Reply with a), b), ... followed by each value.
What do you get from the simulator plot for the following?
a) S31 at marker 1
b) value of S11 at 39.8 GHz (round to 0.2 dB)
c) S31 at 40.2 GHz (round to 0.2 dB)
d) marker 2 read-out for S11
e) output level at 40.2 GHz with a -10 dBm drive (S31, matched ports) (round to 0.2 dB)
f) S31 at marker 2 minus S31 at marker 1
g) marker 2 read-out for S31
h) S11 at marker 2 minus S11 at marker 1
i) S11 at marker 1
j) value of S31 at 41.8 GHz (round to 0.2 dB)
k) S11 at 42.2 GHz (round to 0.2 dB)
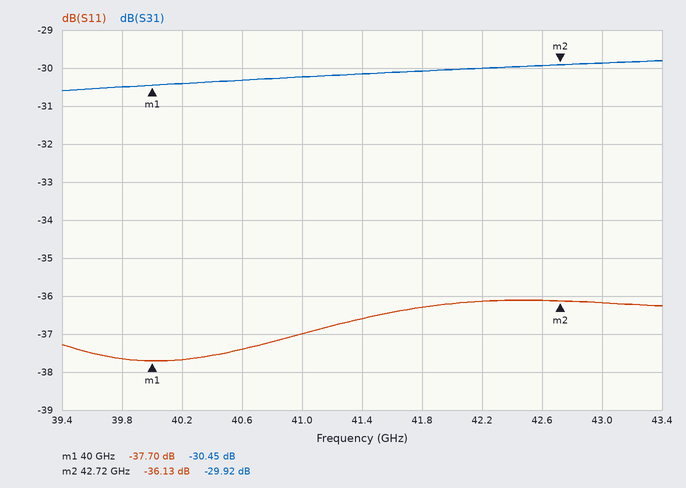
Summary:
a) -30.45 dB
b) -37.6 dB
c) -30.4 dB
d) -36.13 dB
e) -40.4 dBm
f) 0.53 dB
g) -29.92 dB
h) 1.57 dB
i) -37.70 dB
j) -30.0 dB
k) -36.2 dB
